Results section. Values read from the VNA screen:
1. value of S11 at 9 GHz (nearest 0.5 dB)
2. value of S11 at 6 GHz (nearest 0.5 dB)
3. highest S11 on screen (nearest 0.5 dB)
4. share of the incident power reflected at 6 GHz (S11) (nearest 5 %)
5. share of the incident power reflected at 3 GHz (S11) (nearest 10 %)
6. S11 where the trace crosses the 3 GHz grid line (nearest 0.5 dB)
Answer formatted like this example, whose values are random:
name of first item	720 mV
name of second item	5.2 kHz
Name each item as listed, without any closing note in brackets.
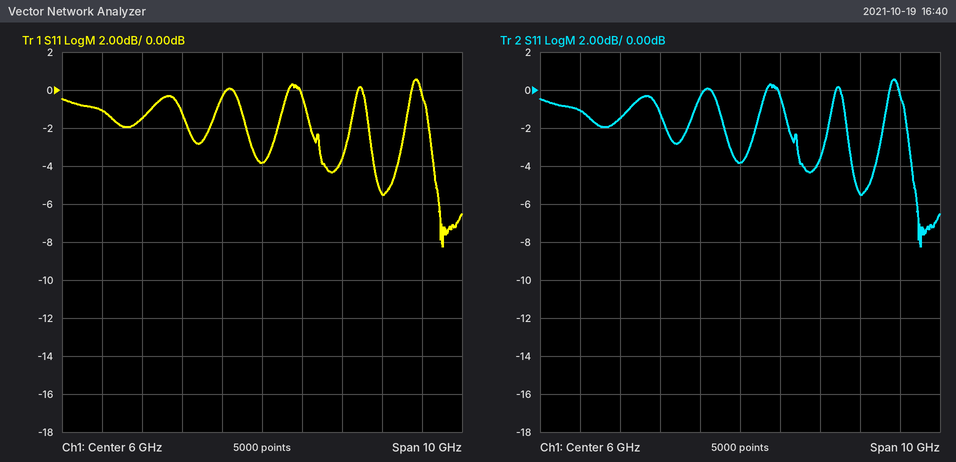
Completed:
value of S11 at 9 GHz	-5.5 dB
value of S11 at 6 GHz	-4.0 dB
highest S11 on screen	0.5 dB
share of the incident power reflected at 6 GHz (S11)	40 %
share of the incident power reflected at 3 GHz (S11)	70 %
S11 where the trace crosses the 3 GHz grid line	-1.5 dB
